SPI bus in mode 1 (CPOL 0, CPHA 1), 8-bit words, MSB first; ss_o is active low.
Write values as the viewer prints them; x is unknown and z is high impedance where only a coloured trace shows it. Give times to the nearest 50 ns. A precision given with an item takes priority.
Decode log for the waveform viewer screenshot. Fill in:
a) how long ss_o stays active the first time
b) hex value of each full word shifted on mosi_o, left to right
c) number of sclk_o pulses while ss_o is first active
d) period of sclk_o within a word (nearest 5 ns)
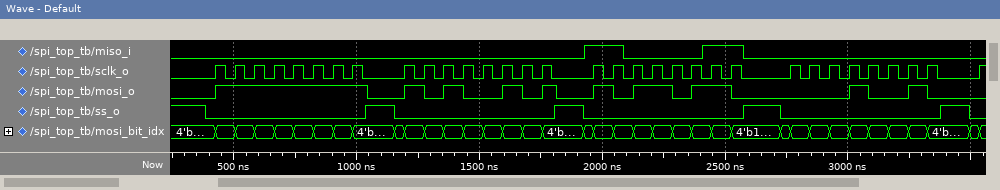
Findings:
650 ns
FF, A5, B6, 12
8
80 ns
